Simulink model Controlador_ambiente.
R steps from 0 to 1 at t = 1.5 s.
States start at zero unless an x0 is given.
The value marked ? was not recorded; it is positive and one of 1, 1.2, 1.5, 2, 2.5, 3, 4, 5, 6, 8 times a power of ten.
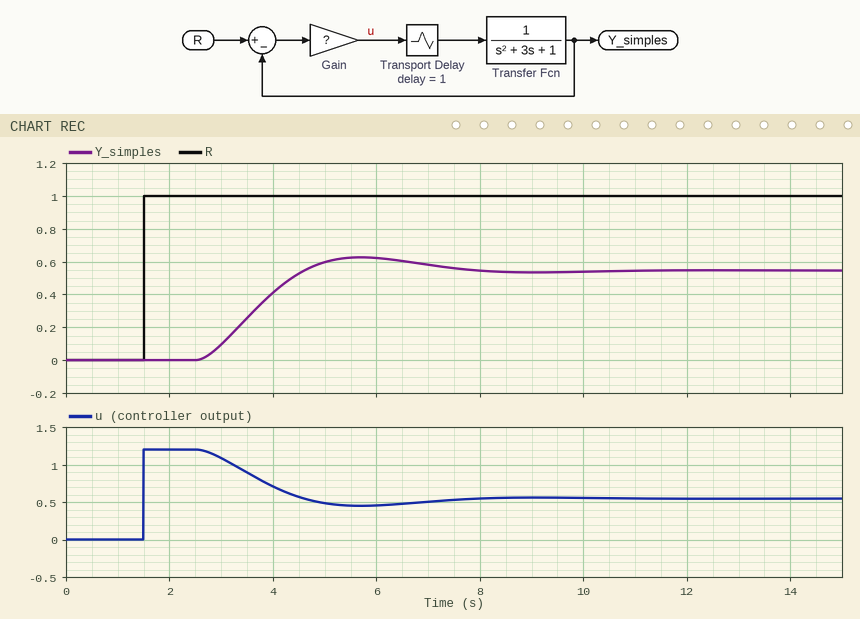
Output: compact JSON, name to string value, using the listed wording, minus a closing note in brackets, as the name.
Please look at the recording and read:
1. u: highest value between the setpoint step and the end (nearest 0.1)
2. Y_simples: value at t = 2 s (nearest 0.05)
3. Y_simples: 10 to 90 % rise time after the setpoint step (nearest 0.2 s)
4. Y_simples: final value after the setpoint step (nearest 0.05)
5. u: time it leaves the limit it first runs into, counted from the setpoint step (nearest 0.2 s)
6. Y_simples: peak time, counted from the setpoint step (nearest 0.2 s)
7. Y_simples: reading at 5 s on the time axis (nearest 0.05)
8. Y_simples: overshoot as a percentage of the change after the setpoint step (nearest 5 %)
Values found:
{"u: highest value between the setpoint step and the end": "1.2", "Y_simples: value at t = 2 s": "0.00", "Y_simples: 10 to 90 % rise time after the setpoint step": "1.4 s", "Y_simples: final value after the setpoint step": "0.55", "u: time it leaves the limit it first runs into, counted from the setpoint step": "1.2 s", "Y_simples: peak time, counted from the setpoint step": "4.2 s", "Y_simples: reading at 5 s on the time axis": "0.60", "Y_simples: overshoot as a percentage of the change after the setpoint step": "15 %"}
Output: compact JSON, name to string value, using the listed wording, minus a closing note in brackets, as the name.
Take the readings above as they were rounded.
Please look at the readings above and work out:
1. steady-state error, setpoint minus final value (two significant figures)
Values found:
{"steady-state error, setpoint minus final value": "0.45"}
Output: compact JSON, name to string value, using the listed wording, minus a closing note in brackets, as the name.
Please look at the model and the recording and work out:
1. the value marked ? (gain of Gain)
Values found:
{"the value marked ?": "1.2"}
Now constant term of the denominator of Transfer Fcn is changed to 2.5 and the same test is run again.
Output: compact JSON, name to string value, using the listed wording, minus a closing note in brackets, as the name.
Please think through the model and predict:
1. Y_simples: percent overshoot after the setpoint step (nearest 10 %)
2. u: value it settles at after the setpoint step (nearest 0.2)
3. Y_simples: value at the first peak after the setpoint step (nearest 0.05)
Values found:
{"Y_simples: percent overshoot after the setpoint step": "20 %", "u: value it settles at after the setpoint step": "0.8", "Y_simples: value at the first peak after the setpoint step": "0.40"}
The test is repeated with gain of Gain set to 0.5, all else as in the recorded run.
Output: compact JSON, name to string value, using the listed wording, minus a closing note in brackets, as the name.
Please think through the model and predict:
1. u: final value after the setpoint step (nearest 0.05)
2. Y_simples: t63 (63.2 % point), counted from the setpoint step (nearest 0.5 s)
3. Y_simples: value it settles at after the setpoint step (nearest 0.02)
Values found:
{"u: final value after the setpoint step": "0.35", "Y_simples: t63 (63.2 % point), counted from the setpoint step": "3.0 s", "Y_simples: value it settles at after the setpoint step": "0.34"}
